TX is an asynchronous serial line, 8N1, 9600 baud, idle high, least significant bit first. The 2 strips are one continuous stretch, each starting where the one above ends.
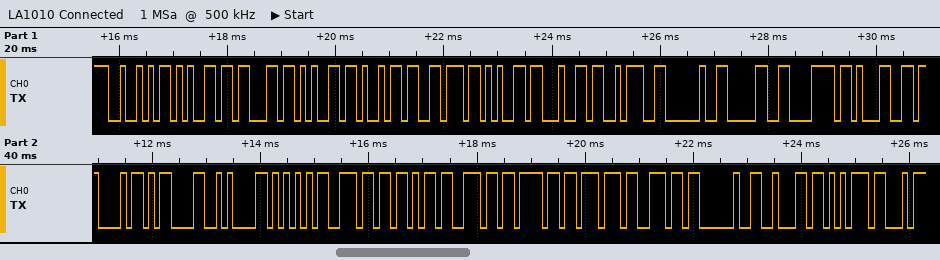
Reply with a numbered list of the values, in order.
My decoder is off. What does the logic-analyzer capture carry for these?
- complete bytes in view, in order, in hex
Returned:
1. 52 65 63 65 69 76 65 64 3A 20 30 78 31 43 0D 0A 55 6E 6B 6E 6F 77 6E 20 62 75
